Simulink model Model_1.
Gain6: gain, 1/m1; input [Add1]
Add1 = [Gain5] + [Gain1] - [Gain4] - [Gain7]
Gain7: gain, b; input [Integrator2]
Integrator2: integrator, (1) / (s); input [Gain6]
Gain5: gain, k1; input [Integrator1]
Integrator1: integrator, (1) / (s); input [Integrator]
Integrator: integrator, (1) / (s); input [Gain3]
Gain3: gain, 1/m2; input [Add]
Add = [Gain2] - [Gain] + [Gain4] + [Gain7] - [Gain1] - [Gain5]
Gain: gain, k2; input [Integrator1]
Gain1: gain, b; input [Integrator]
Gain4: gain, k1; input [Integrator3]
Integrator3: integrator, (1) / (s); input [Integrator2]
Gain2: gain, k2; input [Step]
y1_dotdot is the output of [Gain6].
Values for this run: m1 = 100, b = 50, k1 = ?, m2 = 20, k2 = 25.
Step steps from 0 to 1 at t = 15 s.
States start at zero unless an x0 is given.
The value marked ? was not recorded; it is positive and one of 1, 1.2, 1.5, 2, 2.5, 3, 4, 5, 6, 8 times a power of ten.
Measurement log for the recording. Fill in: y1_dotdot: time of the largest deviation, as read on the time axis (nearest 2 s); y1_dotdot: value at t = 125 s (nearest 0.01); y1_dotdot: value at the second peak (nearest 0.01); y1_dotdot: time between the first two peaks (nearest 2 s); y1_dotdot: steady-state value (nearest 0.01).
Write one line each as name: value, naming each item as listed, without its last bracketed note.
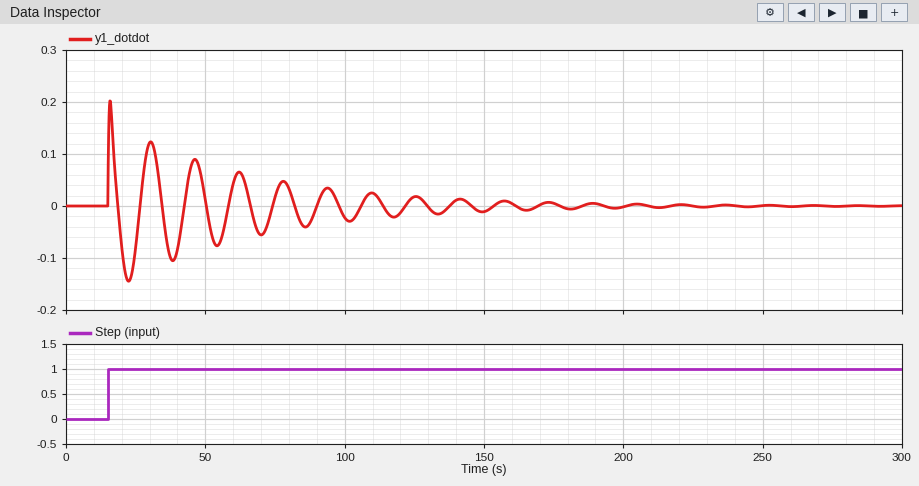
y1_dotdot: time of the largest deviation, as read on the time axis: 16 s
y1_dotdot: value at t = 125 s: 0.02
y1_dotdot: value at the second peak: 0.12
y1_dotdot: time between the first two peaks: 14 s
y1_dotdot: steady-state value: 0.00
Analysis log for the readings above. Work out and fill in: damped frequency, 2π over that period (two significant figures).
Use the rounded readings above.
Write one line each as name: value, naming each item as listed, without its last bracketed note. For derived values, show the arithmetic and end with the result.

damped frequency, 2π over that period: 2π / 14 = 0.45 rad/s
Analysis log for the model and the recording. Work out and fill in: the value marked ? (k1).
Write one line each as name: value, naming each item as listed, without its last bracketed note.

the value marked ?: 50
